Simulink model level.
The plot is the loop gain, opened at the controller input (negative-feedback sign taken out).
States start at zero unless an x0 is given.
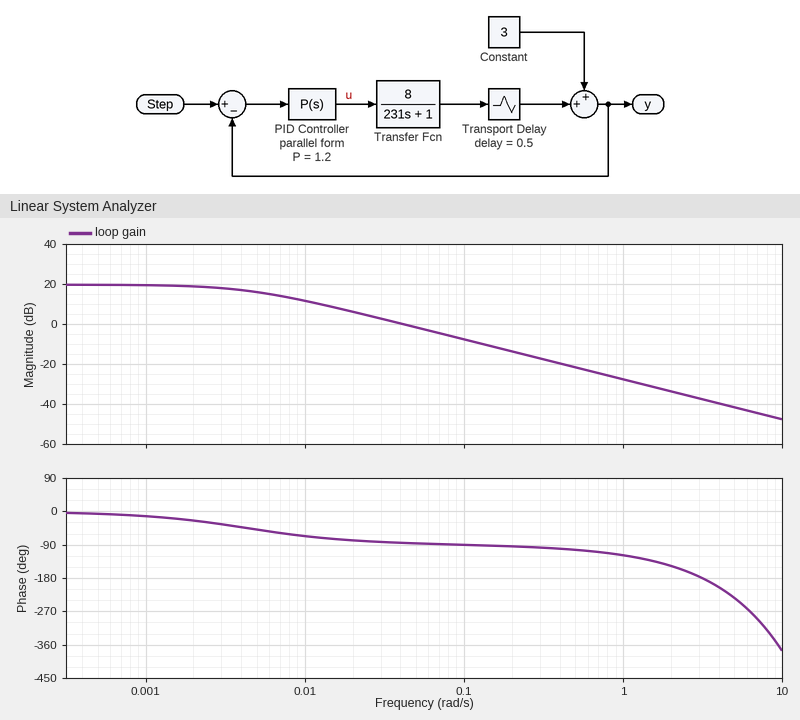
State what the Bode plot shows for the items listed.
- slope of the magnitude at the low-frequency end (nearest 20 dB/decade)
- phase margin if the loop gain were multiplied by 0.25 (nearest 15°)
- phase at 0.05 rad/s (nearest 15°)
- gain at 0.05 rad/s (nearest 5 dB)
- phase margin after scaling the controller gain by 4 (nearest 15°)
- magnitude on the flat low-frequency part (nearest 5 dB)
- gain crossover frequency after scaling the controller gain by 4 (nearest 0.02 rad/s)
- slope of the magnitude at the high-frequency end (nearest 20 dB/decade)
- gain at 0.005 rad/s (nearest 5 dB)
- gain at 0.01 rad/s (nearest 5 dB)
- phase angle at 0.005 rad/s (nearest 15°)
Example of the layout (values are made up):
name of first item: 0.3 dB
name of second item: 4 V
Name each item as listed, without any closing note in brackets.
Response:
slope of the magnitude at the low-frequency end: 0 dB/decade
phase margin if the loop gain were multiplied by 0.25: 120°
phase at 0.05 rad/s: -90°
gain at 0.05 rad/s: 0 dB
phase margin after scaling the controller gain by 4: 90°
magnitude on the flat low-frequency part: 20 dB
gain crossover frequency after scaling the controller gain by 4: 0.16 rad/s
slope of the magnitude at the high-frequency end: -20 dB/decade
gain at 0.005 rad/s: 15 dB
gain at 0.01 rad/s: 10 dB
phase angle at 0.005 rad/s: -45°
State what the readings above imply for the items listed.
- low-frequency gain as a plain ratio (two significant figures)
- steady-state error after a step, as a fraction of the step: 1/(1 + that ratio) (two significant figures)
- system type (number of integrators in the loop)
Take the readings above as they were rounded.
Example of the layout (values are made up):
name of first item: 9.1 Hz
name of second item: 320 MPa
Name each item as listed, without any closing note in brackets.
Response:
low-frequency gain as a plain ratio: 10
steady-state error after a step, as a fraction of the step: 1/(1 + that ratio): 0.091
system type: 0
